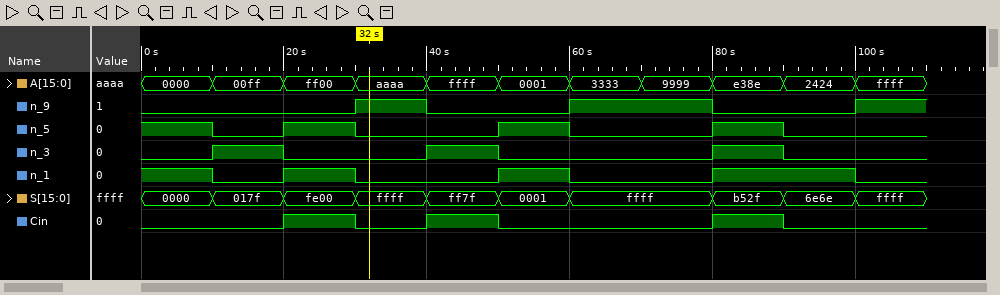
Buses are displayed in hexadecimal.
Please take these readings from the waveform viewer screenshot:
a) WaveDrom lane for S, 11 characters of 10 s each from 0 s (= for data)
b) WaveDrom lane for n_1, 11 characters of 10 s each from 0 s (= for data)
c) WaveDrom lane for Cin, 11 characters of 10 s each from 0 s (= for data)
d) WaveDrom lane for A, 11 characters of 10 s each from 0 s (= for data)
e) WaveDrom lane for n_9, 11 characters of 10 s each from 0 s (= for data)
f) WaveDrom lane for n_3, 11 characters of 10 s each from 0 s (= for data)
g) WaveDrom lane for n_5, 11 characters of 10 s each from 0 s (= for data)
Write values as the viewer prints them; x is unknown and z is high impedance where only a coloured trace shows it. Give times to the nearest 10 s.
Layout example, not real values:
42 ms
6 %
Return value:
{name: 'S', wave: '=======.===', data: '0000 017f fe00 ffff ff7f 0001 ffff b52f 6e6e ffff'}
{name: 'n_1', wave: '1010.10.1.0'}
{name: 'Cin', wave: '0.1010..10.'}
{name: 'A', wave: '===========', data: '0000 00ff ff00 aaaa ffff 0001 3333 9999 e38e 2424 ffff'}
{name: 'n_9', wave: '0..10.1.0.1'}
{name: 'n_3', wave: '010.10..10.'}
{name: 'n_5', wave: '1010.10.10.'}
